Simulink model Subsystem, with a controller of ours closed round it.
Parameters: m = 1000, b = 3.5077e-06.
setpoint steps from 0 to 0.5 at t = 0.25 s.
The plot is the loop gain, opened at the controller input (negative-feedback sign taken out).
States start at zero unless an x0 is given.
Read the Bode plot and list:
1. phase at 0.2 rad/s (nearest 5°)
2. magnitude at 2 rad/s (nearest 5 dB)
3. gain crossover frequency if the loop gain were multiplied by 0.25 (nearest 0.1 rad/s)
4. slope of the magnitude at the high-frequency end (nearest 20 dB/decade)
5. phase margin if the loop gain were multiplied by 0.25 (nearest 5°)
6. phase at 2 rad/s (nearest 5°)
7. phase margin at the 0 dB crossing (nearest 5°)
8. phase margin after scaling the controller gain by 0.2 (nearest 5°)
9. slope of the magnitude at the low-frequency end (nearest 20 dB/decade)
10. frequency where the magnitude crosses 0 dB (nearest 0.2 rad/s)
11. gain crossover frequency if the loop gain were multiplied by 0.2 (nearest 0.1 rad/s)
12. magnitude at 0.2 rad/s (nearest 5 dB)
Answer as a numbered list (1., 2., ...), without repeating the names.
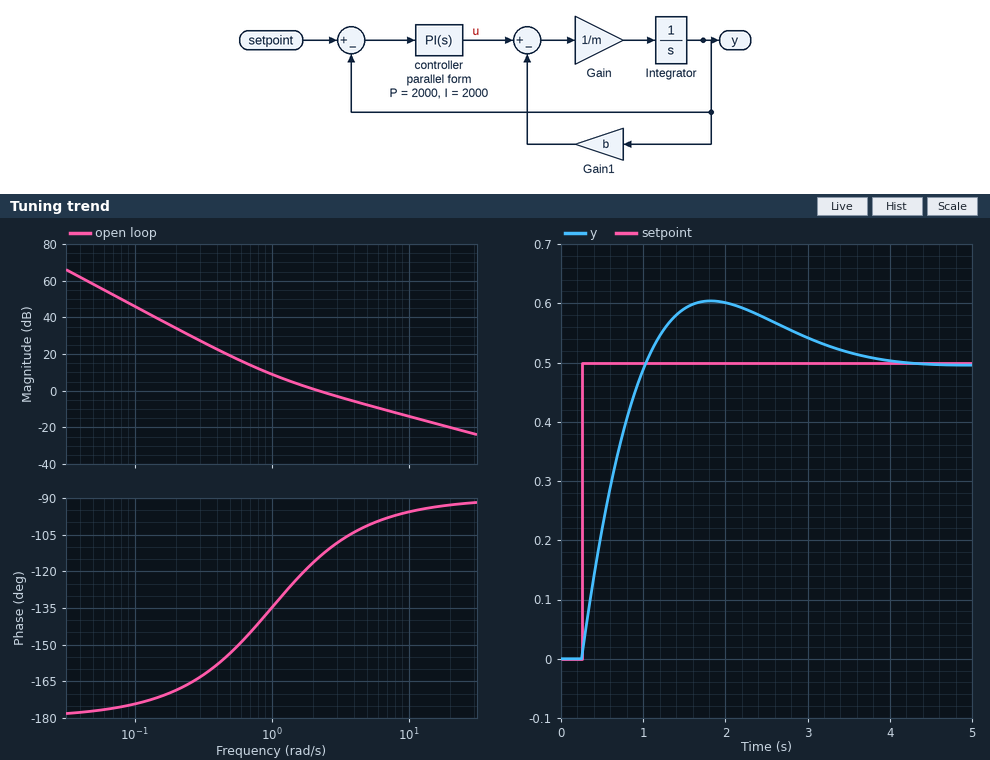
1. -170°
2. 0 dB
3. 0.8 rad/s
4. -20 dB/decade
5. 40°
6. -115°
7. 65°
8. 35°
9. -40 dB/decade
10. 2.2 rad/s
11. 0.7 rad/s
12. 35 dB
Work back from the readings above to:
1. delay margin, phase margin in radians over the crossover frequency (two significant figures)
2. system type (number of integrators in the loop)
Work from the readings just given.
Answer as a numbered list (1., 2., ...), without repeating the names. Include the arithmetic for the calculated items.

1. 65 × π / 180 / 2.2 = 0.52 s
2. 2
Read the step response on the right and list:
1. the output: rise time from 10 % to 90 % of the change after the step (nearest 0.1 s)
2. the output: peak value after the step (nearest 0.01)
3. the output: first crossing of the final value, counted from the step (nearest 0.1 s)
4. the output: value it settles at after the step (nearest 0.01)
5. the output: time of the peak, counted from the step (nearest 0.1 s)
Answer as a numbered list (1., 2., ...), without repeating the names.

1. 0.6 s
2. 0.60
3. 0.8 s
4. 0.50
5. 1.6 s
